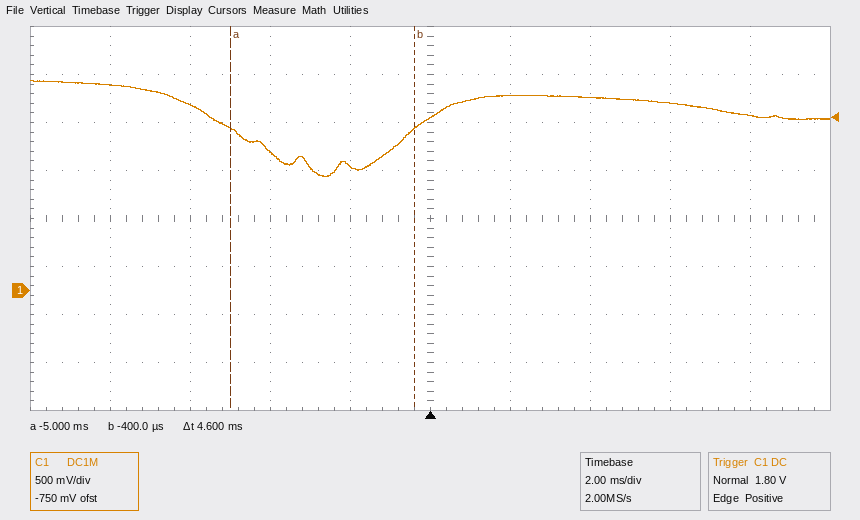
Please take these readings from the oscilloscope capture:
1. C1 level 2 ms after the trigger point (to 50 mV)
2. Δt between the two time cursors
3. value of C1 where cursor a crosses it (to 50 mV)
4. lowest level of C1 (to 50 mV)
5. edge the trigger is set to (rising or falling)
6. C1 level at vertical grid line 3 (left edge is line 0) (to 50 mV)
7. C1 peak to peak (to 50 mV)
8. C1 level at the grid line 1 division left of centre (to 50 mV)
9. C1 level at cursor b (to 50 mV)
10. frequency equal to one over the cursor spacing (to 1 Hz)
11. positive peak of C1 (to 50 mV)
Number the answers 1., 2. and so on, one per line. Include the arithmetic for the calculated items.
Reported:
1. 2.05 V
2. 4.6 ms
3. 1.70 V
4. 1.20 V
5. rising
6. 1.45 V
7. 2.20 V − (1.20 V) = 1.00 V
8. 1.30 V
9. 1.70 V
10. 1 / 4.6 ms ≈ 217 Hz
11. 2.20 V
